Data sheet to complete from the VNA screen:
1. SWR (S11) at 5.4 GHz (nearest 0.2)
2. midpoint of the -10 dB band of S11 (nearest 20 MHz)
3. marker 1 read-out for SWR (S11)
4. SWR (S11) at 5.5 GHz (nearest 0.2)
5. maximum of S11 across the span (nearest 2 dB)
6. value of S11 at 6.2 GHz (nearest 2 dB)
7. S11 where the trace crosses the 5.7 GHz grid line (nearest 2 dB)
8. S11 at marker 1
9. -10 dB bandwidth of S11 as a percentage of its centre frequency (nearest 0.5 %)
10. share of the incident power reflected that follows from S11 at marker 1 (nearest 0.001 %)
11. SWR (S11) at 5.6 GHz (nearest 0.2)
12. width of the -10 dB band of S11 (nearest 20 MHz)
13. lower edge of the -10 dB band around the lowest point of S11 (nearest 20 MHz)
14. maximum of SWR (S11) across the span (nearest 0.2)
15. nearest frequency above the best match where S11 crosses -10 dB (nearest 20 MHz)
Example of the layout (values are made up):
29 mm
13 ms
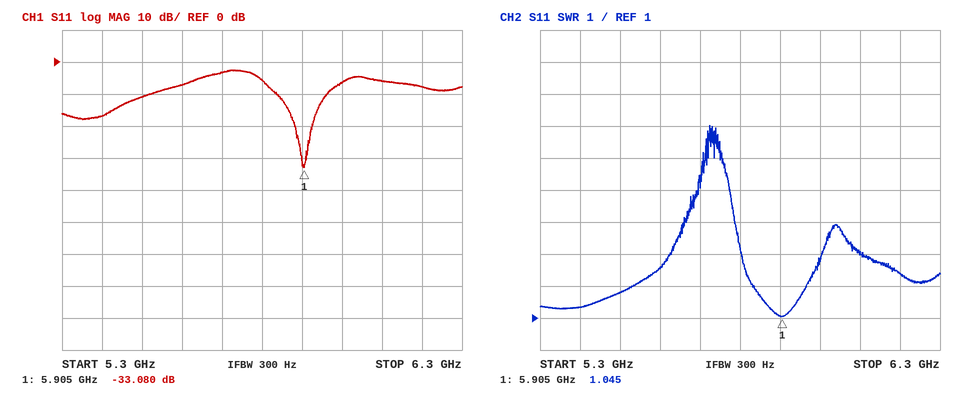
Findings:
1.4
5.90 GHz
1.045
1.8
-2 dB
-8 dB
-4 dB
-33.080 dB
2.0 %
0.049 %
2.6
120 MHz
5.84 GHz
7.0
5.96 GHz
